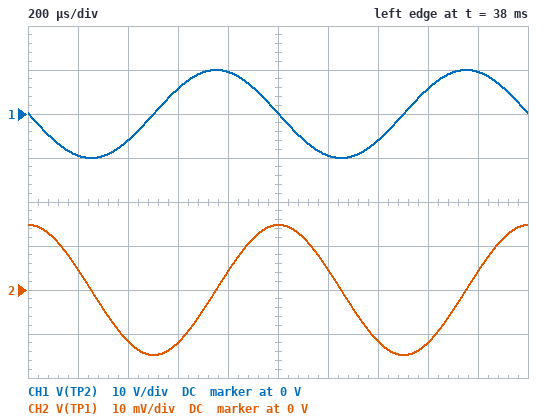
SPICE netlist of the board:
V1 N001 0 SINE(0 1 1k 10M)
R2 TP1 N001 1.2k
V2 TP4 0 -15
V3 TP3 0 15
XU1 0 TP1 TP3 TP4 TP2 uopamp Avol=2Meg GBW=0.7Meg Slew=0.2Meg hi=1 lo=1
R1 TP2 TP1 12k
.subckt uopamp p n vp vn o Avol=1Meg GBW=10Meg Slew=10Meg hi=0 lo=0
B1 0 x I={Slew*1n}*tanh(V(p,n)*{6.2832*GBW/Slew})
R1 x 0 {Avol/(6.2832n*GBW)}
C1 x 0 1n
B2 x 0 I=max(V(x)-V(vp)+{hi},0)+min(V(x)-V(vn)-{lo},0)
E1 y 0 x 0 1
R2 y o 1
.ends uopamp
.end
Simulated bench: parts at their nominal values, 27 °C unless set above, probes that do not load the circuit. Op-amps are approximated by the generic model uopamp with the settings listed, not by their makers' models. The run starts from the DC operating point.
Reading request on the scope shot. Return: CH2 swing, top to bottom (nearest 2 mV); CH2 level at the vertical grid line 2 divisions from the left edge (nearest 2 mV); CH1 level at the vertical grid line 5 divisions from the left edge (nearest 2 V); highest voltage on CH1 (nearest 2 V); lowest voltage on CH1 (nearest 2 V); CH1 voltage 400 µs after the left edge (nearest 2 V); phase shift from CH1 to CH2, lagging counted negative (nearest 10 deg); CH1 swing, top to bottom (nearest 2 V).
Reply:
30 mV
-12 mV
0 V
10 V
-10 V
-6 V
-90 deg
20 V
